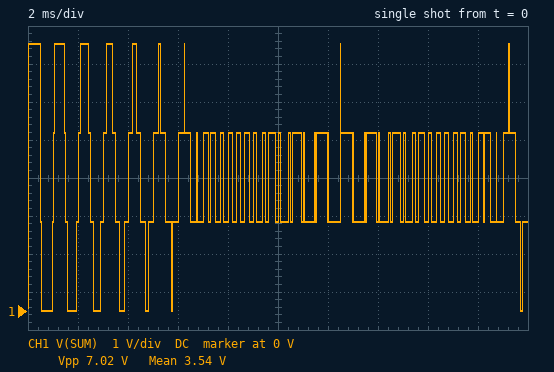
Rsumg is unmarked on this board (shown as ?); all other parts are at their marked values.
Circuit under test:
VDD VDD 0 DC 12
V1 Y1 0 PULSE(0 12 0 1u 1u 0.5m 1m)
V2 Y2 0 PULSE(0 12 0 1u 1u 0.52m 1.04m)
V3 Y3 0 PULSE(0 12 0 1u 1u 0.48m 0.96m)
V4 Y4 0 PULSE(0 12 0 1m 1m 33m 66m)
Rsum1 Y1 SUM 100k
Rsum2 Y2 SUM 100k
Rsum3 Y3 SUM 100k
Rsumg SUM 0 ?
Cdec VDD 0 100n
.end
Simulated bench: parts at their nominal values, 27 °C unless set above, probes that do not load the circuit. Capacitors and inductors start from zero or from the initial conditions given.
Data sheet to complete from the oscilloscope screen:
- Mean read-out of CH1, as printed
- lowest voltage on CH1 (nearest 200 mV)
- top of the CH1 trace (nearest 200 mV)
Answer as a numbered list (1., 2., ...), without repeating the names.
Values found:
1. 3.54 V
2. 0 V
3. 7.0 V
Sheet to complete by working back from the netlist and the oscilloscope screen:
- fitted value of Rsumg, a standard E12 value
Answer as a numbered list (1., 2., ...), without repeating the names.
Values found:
1. 47 kΩ
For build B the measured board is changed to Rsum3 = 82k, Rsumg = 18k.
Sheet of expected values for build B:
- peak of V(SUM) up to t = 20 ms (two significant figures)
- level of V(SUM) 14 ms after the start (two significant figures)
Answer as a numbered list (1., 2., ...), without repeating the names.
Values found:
1. 4.4 V
2. 1.4 V
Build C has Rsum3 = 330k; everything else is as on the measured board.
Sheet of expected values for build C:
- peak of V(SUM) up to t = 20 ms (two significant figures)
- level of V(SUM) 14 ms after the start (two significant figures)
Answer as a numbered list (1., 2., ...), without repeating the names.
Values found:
1. 6.2 V
2. 2.7 V
